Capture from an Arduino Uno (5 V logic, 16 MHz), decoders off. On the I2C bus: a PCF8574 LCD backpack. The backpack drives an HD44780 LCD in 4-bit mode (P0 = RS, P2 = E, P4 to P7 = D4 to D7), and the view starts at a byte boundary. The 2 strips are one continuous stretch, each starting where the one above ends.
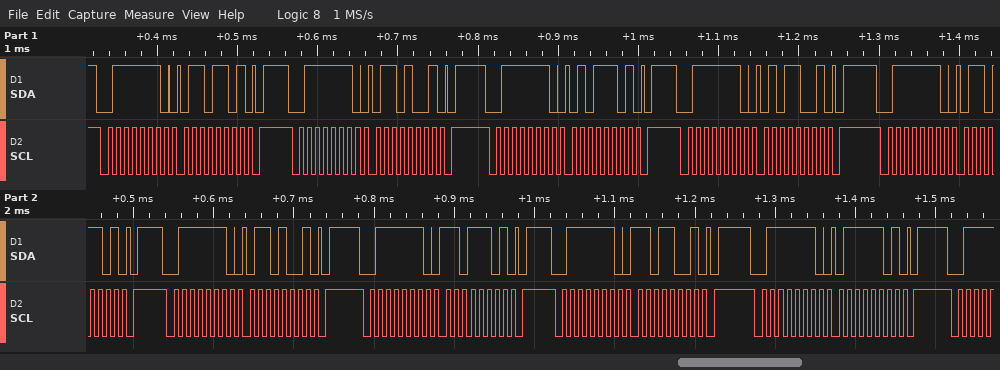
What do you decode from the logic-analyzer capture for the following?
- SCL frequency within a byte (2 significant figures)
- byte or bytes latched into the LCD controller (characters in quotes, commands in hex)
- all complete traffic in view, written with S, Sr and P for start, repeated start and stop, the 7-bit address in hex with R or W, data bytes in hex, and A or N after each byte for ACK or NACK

100 kHz
'e' 'm'
S 3FW A 6D A P S 3FW A 69 A P S 3FW A 5D A P S 3FW A 59 A P S 3FW A 6D A P S 3FW A 69 A P S 3FW A DD A P S 3FW A D9 A P S 3FW A 7D A P
